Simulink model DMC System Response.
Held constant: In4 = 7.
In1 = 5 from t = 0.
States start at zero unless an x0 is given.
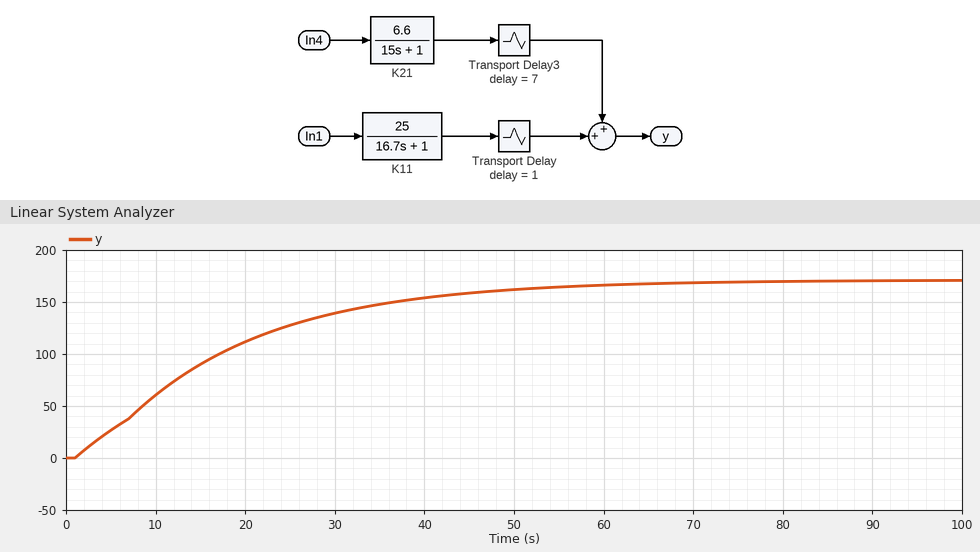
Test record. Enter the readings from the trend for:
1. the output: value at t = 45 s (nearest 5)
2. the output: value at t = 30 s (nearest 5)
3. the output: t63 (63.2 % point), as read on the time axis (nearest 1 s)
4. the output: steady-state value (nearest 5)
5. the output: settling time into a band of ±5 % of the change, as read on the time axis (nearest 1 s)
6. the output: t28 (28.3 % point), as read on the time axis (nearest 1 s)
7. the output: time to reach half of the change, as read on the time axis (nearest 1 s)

160
140
19 s
170
51 s
8 s
14 s
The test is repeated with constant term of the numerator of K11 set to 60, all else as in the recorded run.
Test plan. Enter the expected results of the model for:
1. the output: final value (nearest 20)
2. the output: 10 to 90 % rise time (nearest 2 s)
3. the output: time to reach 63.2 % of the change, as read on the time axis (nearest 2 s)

340
36 s
18 s
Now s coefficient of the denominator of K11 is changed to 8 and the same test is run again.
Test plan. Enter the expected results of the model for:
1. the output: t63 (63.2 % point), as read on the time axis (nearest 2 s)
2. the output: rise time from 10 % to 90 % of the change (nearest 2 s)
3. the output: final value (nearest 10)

12 s
24 s
170
